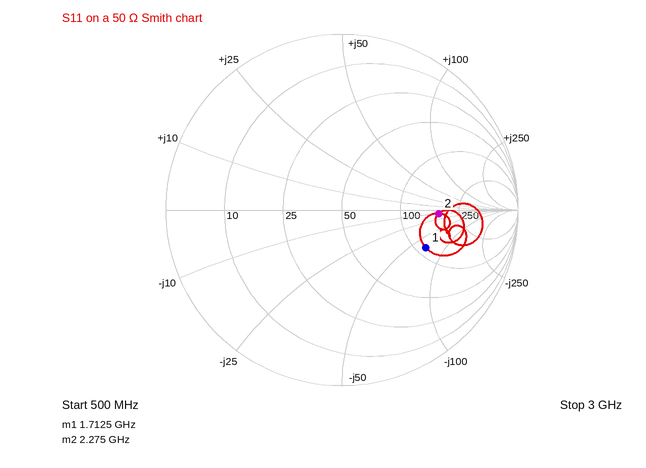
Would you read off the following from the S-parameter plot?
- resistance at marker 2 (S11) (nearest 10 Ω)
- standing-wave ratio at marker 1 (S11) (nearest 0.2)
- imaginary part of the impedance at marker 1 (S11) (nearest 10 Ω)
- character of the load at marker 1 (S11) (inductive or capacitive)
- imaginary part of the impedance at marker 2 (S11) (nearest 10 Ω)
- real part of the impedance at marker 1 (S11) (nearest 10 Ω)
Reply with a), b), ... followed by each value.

a) 170 Ω
b) 3.2
c) -70 Ω
d) capacitive
e) -10 Ω
f) 110 Ω
